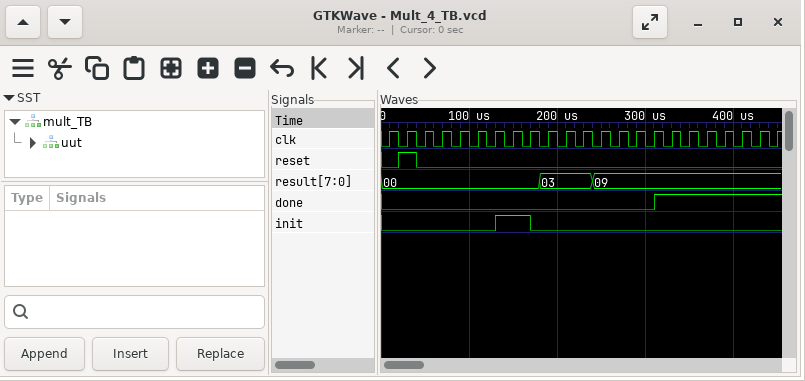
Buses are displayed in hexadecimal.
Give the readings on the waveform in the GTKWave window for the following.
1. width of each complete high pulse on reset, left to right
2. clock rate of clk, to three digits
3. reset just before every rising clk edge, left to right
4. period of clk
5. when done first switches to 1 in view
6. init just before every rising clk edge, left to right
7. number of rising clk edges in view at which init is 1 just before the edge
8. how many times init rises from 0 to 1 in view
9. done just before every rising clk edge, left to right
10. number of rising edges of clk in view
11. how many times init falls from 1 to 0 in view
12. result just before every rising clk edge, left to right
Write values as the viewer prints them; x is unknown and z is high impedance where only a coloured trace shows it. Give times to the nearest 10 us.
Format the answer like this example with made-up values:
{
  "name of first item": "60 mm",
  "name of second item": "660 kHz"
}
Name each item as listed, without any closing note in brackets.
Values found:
{
  "width of each complete high pulse on reset, left to right": "20 us",
  "clock rate of clk, to three digits": "50.0 kHz",
  "reset just before every rising clk edge, left to right": "0 1 0 0 0 0 0 0 0 0 0 0 0 0 0 0 0 0 0 0 0 0 0",
  "period of clk": "20 us",
  "when done first switches to 1 in view": "310 us",
  "init just before every rising clk edge, left to right": "0 0 0 0 0 0 0 1 1 0 0 0 0 0 0 0 0 0 0 0 0 0 0",
  "number of rising clk edges in view at which init is 1 just before the edge": "2",
  "how many times init rises from 0 to 1 in view": "1",
  "done just before every rising clk edge, left to right": "0 0 0 0 0 0 0 0 0 0 0 0 0 0 0 0 1 1 1 1 1 1 1",
  "number of rising edges of clk in view": "23",
  "how many times init falls from 1 to 0 in view": "1",
  "result just before every rising clk edge, left to right": "00, 00, 00, 00, 00, 00, 00, 00, 00, 03, 03, 03, 09, 09, 09, 09, 09, 09, 09, 09, 09, 09, 09"
}
